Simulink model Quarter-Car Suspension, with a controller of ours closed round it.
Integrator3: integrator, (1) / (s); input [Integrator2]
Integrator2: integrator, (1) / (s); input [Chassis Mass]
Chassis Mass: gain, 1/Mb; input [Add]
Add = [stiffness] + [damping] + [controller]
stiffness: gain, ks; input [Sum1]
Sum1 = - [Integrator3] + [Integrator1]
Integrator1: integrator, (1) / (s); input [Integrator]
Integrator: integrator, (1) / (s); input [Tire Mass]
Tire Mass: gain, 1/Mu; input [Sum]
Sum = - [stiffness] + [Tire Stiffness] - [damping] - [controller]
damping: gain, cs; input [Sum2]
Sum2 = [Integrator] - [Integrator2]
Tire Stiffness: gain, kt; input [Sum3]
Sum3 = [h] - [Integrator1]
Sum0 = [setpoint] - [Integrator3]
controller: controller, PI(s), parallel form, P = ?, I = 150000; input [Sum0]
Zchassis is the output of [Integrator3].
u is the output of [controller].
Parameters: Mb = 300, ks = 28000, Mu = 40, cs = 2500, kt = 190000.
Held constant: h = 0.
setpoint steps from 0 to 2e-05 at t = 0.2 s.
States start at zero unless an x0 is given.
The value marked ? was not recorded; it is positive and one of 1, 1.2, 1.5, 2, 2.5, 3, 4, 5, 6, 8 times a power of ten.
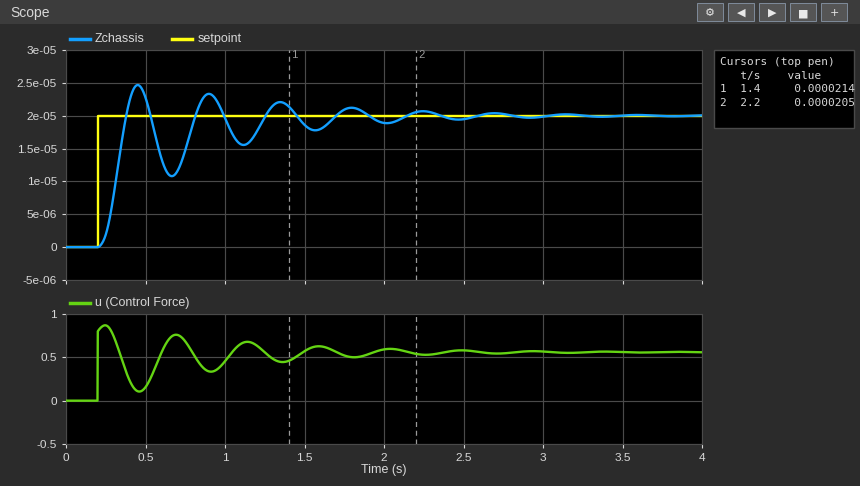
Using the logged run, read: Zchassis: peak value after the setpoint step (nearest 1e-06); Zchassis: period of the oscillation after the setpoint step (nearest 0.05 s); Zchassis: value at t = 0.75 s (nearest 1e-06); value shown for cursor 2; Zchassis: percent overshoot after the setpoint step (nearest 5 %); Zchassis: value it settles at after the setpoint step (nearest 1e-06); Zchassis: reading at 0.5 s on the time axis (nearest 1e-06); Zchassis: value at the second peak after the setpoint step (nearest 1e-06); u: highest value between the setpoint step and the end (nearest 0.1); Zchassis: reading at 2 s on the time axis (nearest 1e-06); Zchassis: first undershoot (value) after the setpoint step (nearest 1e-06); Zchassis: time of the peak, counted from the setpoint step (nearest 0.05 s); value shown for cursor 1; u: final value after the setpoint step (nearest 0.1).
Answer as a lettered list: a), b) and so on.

a) 0.000025
b) 0.45 s
c) 0.000015
d) 0.0000205
e) 25 %
f) 0.000020
g) 0.000023
h) 0.000023
i) 0.9
j) 0.000019
k) 0.000011
l) 0.25 s
m) 0.0000214
n) 0.6
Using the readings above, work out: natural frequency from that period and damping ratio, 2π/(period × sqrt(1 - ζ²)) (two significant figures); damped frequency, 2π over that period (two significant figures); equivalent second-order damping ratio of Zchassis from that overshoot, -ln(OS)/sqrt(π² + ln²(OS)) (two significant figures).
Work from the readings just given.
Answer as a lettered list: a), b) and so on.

a) 15 rad/s
b) 14 rad/s
c) 0.40
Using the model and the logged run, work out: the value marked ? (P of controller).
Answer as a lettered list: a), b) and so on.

a) 40000
